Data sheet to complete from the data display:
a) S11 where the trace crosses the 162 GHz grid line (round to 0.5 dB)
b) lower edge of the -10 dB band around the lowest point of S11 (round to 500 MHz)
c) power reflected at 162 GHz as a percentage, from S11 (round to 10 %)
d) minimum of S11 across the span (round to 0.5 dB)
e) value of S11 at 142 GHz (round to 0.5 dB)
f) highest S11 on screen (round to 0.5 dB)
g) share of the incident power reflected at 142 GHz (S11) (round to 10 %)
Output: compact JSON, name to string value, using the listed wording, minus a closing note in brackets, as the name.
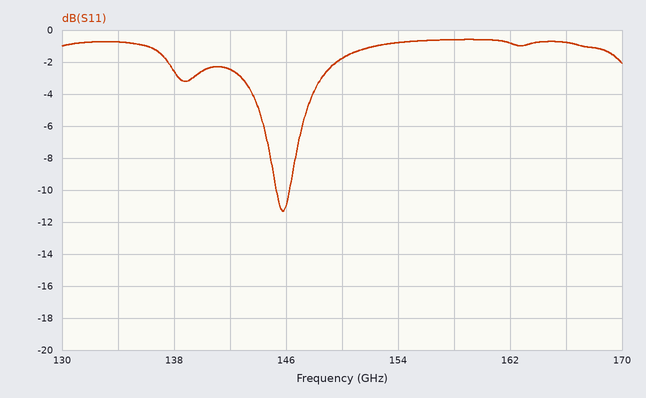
{"S11 where the trace crosses the 162 GHz grid line": "-1.0 dB", "lower edge of the -10 dB band around the lowest point of S11": "145.5 GHz", "power reflected at 162 GHz as a percentage, from S11": "80 %", "minimum of S11 across the span": "-11.5 dB", "value of S11 at 142 GHz": "-2.5 dB", "highest S11 on screen": "-0.5 dB", "share of the incident power reflected at 142 GHz (S11)": "60 %"}
